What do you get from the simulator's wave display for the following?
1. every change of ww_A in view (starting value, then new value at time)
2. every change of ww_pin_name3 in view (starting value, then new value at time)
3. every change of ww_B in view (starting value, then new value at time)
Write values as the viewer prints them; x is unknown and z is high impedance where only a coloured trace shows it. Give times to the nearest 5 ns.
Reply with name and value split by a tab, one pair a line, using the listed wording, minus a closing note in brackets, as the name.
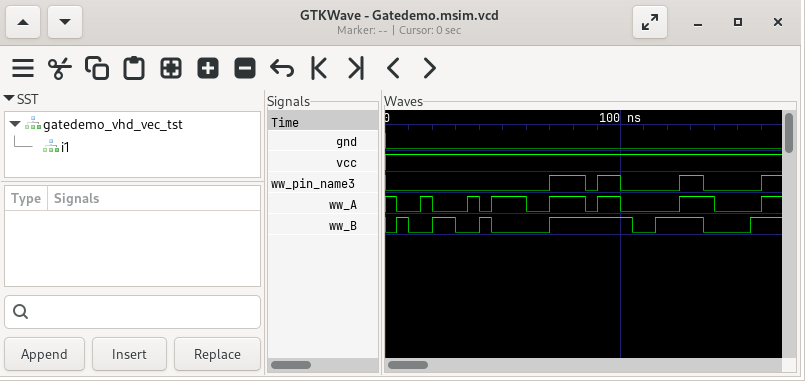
every change of ww_A in view	1, 0 at 5 ns, 1 at 15 ns, 0 at 20 ns, 1 at 35 ns, 0 at 40 ns, 1 at 45 ns, 0 at 60 ns, 1 at 70 ns, 0 at 85 ns, 1 at 90 ns, 0 at 100 ns, 1 at 125 ns, 0 at 140 ns, 1 at 160 ns
every change of ww_pin_name3 in view	0, 1 at 70 ns, 0 at 85 ns, 1 at 90 ns, 0 at 100 ns, 1 at 125 ns, 0 at 135 ns, 1 at 160 ns
every change of ww_B in view	0, 1 at 5 ns, 0 at 10 ns, 1 at 20 ns, 0 at 30 ns, 1 at 40 ns, 0 at 45 ns, 1 at 70 ns, 0 at 105 ns, 1 at 115 ns, 0 at 135 ns, 1 at 155 ns
